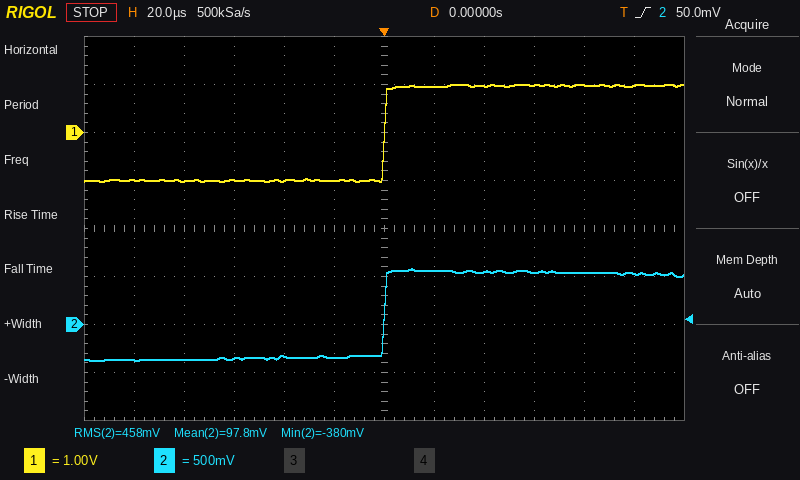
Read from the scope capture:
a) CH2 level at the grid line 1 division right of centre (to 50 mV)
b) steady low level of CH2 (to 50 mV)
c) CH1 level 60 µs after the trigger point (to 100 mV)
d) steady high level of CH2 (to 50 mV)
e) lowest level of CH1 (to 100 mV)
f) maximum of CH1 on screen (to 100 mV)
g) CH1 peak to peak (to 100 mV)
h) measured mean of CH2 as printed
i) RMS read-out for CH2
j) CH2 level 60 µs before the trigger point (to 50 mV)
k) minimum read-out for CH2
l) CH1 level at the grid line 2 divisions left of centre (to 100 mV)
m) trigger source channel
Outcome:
550 mV
-350 mV
1.0 V
550 mV
-1.0 V
1.0 V
2.0 V
97.8 mV
458 mV
-350 mV
-380 mV
-1.0 V
CH2
